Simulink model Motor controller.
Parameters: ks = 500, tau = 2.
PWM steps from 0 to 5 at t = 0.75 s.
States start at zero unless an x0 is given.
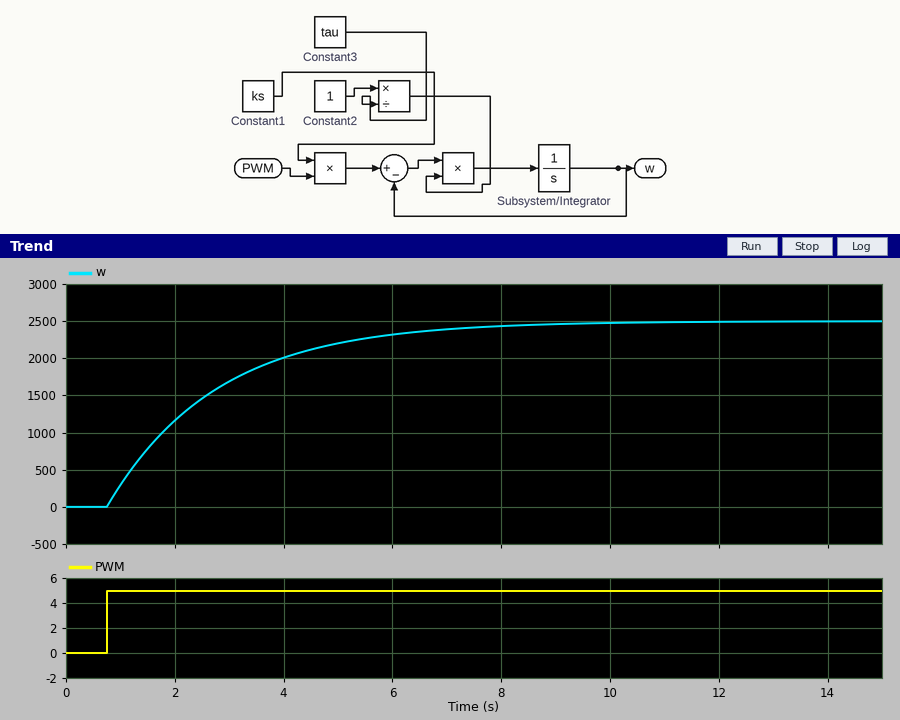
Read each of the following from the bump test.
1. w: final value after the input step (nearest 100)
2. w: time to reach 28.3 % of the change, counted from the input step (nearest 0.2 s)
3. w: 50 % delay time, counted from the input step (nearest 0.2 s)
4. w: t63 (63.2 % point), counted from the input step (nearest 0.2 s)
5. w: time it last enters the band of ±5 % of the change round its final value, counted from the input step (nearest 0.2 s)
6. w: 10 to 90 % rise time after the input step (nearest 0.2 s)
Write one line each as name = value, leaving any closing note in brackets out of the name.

w: final value after the input step = 2500
w: time to reach 28.3 % of the change, counted from the input step = 0.6 s
w: 50 % delay time, counted from the input step = 1.4 s
w: t63 (63.2 % point), counted from the input step = 2.0 s
w: time it last enters the band of ±5 % of the change round its final value, counted from the input step = 6.0 s
w: 10 to 90 % rise time after the input step = 4.4 s
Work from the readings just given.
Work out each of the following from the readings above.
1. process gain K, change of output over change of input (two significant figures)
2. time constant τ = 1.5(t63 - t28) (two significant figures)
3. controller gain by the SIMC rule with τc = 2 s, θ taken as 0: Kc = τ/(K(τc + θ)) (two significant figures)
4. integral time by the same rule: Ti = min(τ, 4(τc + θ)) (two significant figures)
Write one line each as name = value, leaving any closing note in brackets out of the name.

process gain K, change of output over change of input = 500
time constant τ = 1.5(t63 - t28) = 2.1 s
controller gain by the SIMC rule with τc = 2 s, θ taken as 0: Kc = τ/(K(τc + θ)) = 0.0021
integral time by the same rule: Ti = min(τ, 4(τc + θ)) = 2.1 s
